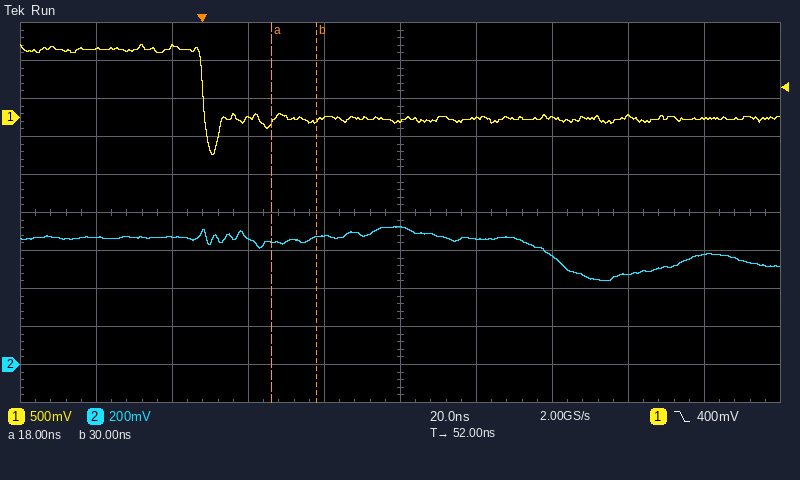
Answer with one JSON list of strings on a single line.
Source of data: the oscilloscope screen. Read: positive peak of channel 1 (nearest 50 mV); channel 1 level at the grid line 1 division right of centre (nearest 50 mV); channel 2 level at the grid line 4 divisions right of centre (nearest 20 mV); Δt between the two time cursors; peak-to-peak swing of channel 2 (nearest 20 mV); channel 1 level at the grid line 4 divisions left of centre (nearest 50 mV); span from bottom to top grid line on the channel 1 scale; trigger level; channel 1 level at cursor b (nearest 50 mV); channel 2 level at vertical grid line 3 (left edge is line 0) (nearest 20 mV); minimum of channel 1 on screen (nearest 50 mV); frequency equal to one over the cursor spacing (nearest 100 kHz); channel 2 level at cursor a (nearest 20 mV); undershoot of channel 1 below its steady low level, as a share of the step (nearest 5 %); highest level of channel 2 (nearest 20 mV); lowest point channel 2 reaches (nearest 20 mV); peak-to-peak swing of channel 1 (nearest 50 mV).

["950 mV", "0 mV", "580 mV", "12 ns", "280 mV", "900 mV", "5 V", "400 mV", "-50 mV", "660 mV", "-500 mV", "83.3 MHz", "640 mV", "50 %", "720 mV", "440 mV", "1.45 V"]
